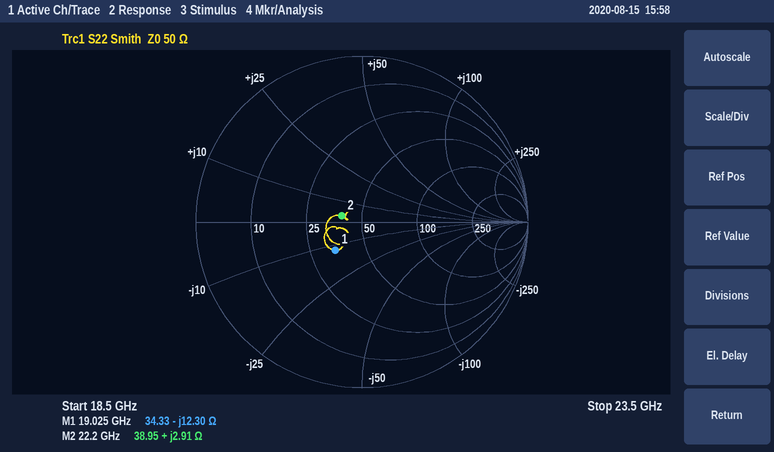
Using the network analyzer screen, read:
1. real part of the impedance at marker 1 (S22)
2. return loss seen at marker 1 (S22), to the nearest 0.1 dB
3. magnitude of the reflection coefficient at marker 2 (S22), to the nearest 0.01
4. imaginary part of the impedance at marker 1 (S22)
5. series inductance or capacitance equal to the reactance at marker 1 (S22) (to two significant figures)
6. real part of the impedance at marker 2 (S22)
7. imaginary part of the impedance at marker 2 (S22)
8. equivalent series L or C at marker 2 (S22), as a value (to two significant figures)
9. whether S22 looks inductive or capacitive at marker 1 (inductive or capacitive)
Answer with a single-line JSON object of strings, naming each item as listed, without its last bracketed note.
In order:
{"real part of the impedance at marker 1": "34.33 Ω", "return loss seen at marker 1 (S22), to the nearest 0.1 dB": "12.6 dB", "magnitude of the reflection coefficient at marker 2 (S22), to the nearest 0.01": "0.13", "imaginary part of the impedance at marker 1": "-12.30 Ω", "series inductance or capacitance equal to the reactance at marker 1 (S22)": "680 fF", "real part of the impedance at marker 2": "38.95 Ω", "imaginary part of the impedance at marker 2": "+2.91 Ω", "equivalent series L or C at marker 2 (S22), as a value": "21 pH", "whether S22 looks inductive or capacitive at marker 1": "capacitive"}
